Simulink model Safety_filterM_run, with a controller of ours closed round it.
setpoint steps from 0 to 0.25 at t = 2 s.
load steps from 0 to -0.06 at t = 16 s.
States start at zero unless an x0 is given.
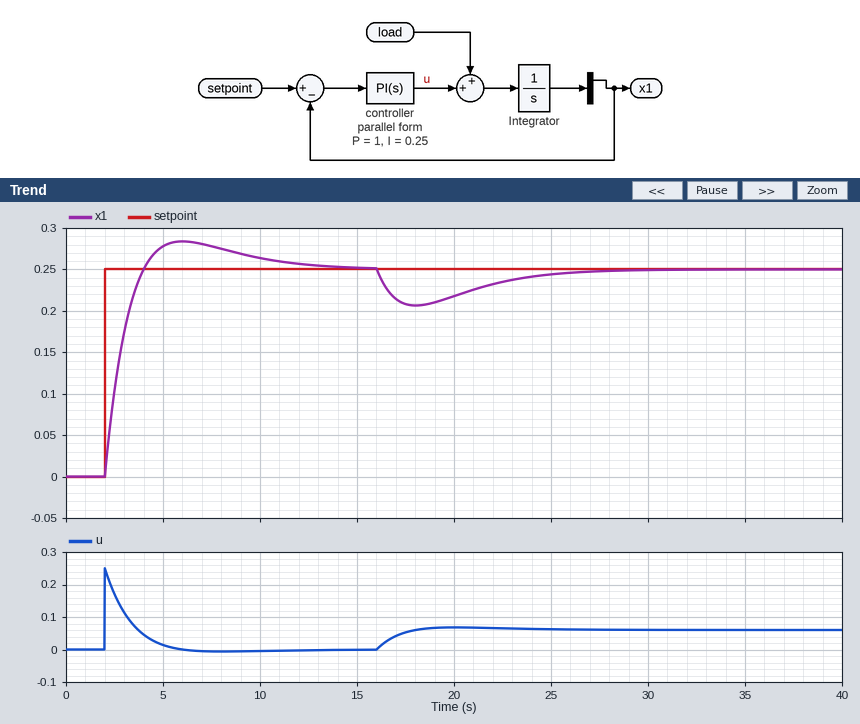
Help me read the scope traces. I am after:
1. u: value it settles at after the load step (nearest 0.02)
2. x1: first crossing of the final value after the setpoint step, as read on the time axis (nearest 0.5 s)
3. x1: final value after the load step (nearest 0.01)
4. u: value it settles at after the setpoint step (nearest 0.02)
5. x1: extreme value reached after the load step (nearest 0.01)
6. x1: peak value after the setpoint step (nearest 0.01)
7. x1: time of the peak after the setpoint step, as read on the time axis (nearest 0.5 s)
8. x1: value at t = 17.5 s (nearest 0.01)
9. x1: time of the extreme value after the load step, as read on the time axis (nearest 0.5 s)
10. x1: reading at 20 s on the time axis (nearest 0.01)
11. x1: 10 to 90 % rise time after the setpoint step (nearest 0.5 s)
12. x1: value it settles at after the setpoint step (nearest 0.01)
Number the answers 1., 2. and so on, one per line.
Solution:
1. 0.06
2. 4.0 s
3. 0.25
4. 0.00
5. 0.21
6. 0.28
7. 6.0 s
8. 0.21
9. 18.0 s
10. 0.22
11. 1.5 s
12. 0.25
